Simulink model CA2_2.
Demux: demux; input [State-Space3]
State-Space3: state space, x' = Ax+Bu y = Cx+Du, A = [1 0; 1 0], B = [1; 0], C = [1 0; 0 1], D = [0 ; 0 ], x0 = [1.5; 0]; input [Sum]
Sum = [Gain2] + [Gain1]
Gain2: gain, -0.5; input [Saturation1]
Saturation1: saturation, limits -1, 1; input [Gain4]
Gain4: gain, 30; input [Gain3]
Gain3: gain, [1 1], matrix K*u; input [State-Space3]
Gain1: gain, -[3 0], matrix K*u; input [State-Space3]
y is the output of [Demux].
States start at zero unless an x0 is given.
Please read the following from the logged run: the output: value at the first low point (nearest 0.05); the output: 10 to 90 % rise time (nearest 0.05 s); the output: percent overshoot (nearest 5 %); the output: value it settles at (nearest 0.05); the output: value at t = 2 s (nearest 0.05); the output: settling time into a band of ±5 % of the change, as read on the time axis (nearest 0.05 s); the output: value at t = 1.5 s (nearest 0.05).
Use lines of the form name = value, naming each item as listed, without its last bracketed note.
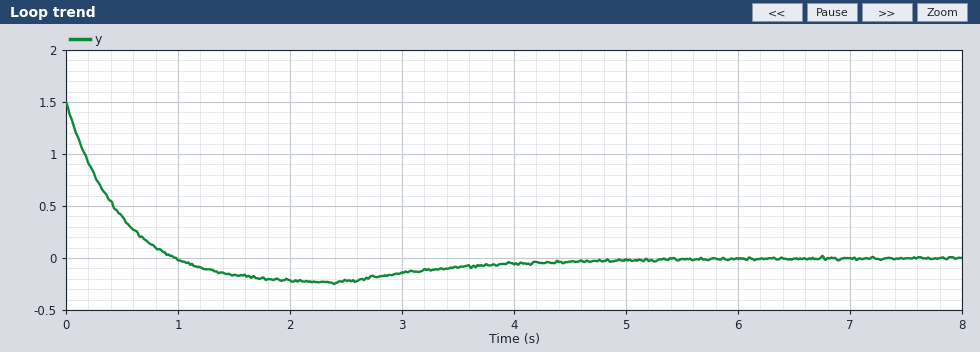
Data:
the output: value at the first low point = -0.25
the output: 10 to 90 % rise time = 0.70 s
the output: percent overshoot = 15 %
the output: value it settles at = 0.00
the output: value at t = 2 s = -0.20
the output: settling time into a band of ±5 % of the change, as read on the time axis = 3.70 s
the output: value at t = 1.5 s = -0.15
